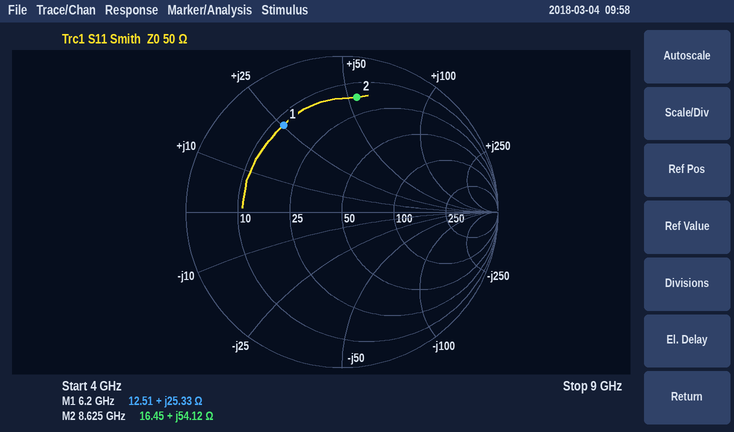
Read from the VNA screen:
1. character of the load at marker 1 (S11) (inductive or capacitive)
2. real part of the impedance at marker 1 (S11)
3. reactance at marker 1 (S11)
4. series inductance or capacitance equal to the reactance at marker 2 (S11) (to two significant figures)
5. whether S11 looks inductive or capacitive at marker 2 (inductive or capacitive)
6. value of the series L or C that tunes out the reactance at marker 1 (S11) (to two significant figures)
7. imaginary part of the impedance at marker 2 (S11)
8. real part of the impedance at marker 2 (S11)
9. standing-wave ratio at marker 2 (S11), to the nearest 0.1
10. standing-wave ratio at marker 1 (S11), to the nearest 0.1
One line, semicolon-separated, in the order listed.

inductive; 12.51 Ω; +25.33 Ω; 1.00 nH; inductive; 1.0 pF; +54.12 Ω; 16.45 Ω; 6.8; 5.1
